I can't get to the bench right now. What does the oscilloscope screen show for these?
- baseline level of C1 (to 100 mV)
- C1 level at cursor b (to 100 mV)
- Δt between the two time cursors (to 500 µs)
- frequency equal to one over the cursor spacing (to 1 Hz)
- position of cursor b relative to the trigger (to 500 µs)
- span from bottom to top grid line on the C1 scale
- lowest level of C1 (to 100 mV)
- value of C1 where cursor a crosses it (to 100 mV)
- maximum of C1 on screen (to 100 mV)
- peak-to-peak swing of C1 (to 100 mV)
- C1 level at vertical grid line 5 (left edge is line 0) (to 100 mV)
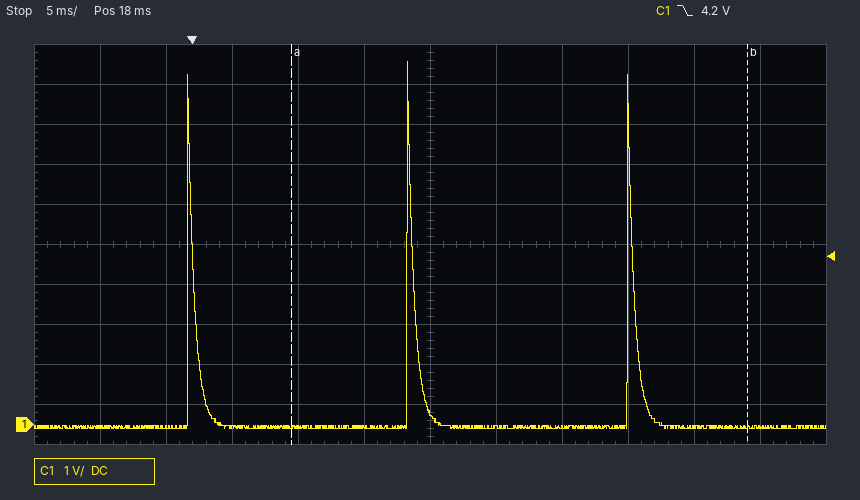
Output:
-100 mV
-100 mV
34.5 ms
29 Hz
+42.0 ms
10 V
-100 mV
-100 mV
9.1 V
9.2 V
-100 mV
